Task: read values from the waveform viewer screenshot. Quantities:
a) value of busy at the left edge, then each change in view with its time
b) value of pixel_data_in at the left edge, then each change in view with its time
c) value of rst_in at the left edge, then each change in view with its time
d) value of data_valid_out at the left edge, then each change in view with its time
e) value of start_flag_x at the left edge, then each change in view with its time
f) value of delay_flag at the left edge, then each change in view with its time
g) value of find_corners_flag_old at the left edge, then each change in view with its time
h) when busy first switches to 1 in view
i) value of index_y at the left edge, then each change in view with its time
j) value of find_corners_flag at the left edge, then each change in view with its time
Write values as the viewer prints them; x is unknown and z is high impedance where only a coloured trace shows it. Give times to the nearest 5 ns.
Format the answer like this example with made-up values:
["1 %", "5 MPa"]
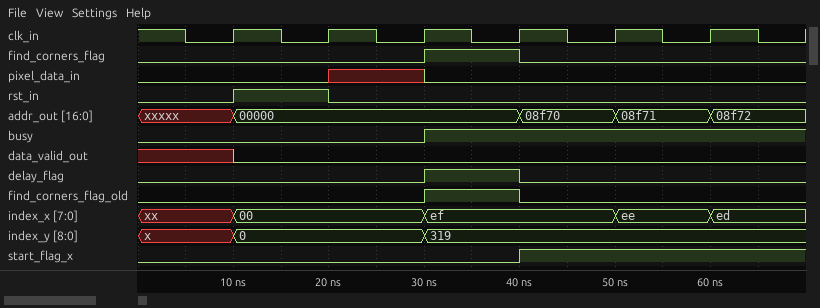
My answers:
["0, 1 at 30 ns", "0, x at 20 ns, 0 at 30 ns", "0, 1 at 10 ns, 0 at 20 ns", "x, 0 at 10 ns", "0, 1 at 40 ns", "0, 1 at 30 ns, 0 at 40 ns", "0, 1 at 30 ns, 0 at 40 ns", "30 ns", "x, 0 at 10 ns, 319 at 30 ns", "0, 1 at 30 ns, 0 at 40 ns"]
